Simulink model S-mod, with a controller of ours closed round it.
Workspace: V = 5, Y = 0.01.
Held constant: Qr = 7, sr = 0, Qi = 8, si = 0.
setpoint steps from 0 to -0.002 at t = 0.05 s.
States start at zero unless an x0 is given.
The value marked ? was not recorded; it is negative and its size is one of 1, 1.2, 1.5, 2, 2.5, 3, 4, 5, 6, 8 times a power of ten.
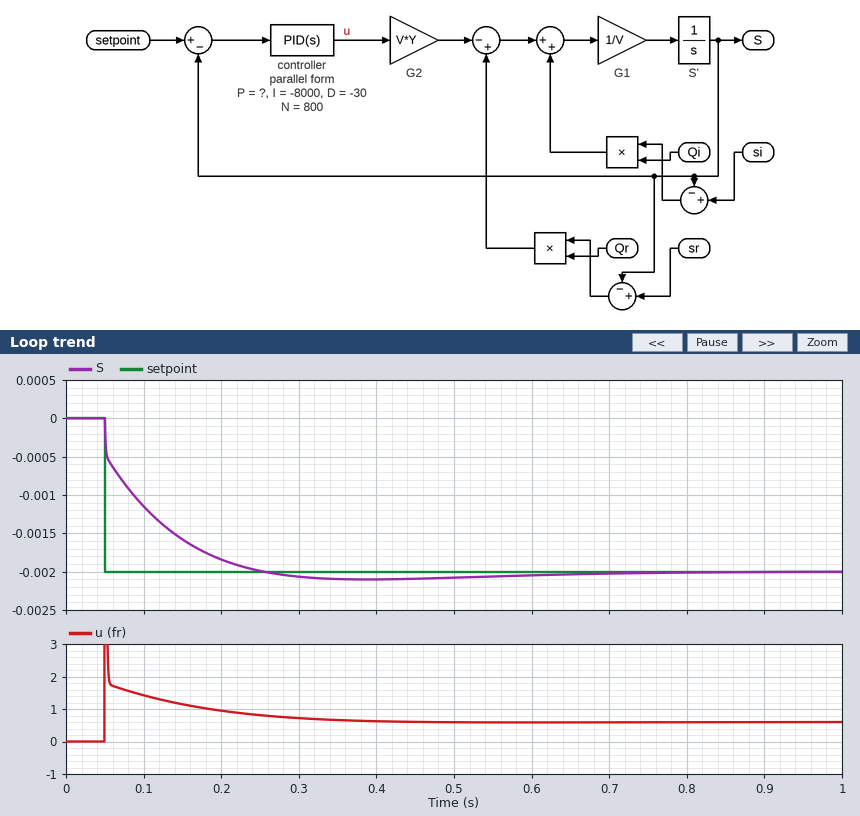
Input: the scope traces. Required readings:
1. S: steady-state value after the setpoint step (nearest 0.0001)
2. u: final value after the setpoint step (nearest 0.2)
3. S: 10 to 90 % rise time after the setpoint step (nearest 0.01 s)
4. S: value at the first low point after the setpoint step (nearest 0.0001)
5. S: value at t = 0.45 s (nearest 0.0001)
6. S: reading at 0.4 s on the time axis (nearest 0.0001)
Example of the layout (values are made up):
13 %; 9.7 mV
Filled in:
-0.0020; 0.6; 0.14 s; -0.0021; -0.0021; -0.0021
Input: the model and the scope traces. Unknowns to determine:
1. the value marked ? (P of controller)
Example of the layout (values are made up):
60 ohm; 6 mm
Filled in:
-1500
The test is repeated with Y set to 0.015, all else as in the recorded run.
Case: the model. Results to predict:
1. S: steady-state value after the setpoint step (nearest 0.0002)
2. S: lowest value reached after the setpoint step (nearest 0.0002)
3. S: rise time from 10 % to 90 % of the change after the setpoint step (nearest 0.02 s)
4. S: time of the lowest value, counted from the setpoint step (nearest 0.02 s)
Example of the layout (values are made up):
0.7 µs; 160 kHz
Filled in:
-0.0020; -0.0020; 0.10 s; 0.28 s
